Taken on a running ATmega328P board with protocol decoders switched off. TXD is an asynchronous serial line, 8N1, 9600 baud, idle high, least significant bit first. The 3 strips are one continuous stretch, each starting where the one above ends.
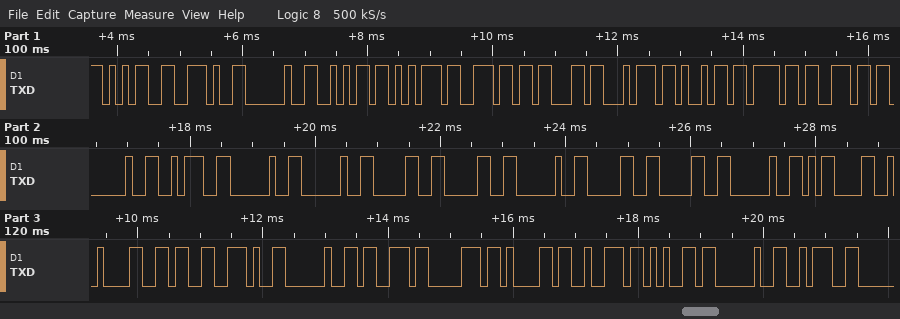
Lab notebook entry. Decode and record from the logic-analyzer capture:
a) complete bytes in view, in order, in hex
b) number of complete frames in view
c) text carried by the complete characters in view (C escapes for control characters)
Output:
35 2E 20 6A 75 6E 63 74 69 6F 6E 20 3A 20 20 30 30 20 30 30 20 0D 0A 36 2E 20 73 70 61 72 65 20 3A
33
"5. junction :  00 00 \r\n6. spare :"
